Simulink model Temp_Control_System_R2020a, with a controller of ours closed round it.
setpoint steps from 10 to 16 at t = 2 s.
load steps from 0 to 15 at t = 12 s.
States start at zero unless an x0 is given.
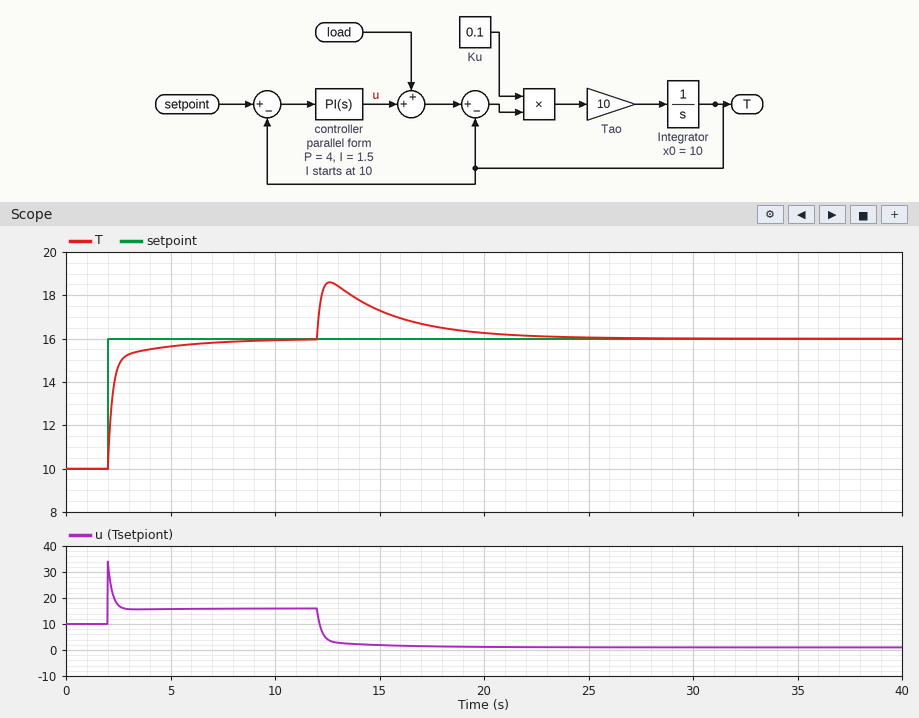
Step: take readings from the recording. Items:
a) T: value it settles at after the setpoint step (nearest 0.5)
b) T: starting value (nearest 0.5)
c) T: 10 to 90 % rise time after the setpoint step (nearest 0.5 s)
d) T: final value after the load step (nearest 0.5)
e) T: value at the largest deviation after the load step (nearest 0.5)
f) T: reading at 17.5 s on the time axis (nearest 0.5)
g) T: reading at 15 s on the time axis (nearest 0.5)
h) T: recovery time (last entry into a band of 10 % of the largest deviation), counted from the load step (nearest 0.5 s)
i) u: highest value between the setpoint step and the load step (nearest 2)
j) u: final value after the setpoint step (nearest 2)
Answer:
16.0
10.0
1.5 s
16.0
18.5
16.5
17.5
8.0 s
34
16
